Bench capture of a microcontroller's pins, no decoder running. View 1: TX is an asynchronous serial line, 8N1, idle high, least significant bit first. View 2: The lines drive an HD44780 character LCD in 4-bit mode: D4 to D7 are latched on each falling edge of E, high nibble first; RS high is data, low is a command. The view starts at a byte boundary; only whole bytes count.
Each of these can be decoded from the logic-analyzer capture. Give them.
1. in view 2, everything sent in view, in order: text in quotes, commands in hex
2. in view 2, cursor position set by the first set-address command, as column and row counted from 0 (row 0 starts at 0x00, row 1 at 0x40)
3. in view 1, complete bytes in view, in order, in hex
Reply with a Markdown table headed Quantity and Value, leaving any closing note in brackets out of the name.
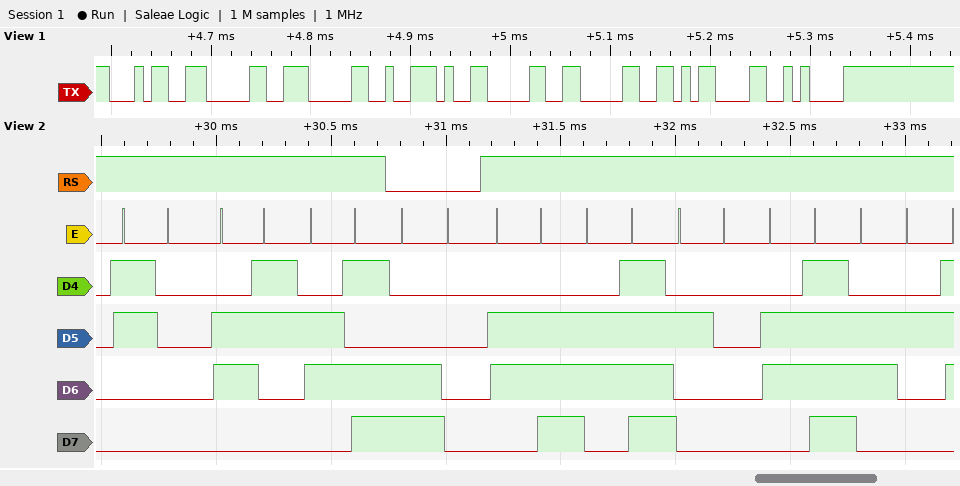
| Quantity | Value |
|---|---|
| in view 2, everything sent in view, in order: text in quotes, commands in hex | "0cm" 0xC0 "no ob" |
| in view 2, cursor position set by the first set-address command, as column and row counted from 0 | column 0, row 1 |
| in view 1, complete bytes in view, in order, in hex | 34 30 30 2E 30 30 0D 0A |
